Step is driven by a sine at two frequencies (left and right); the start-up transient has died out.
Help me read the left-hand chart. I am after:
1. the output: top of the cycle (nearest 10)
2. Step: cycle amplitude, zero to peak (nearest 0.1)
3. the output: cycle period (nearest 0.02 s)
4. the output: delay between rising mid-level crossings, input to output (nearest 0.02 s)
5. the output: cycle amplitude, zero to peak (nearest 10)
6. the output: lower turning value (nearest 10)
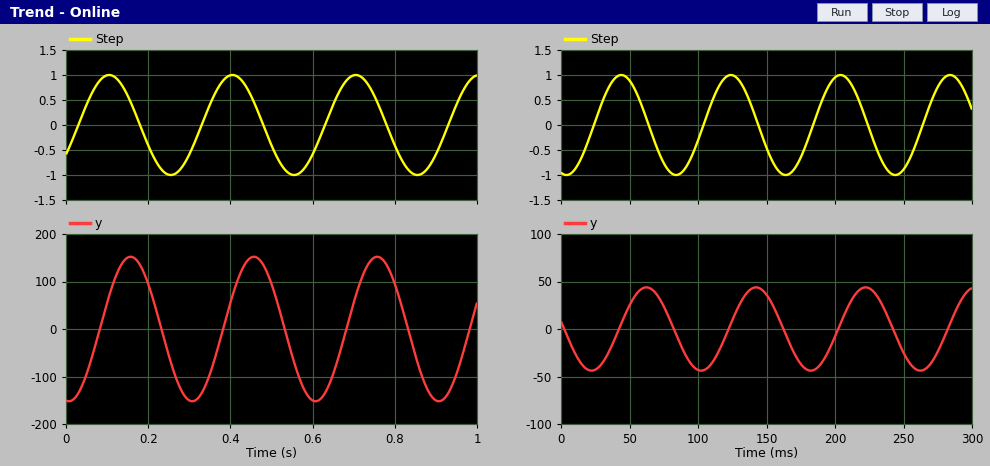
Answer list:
150
1.0
0.30 s
0.06 s
150
-150
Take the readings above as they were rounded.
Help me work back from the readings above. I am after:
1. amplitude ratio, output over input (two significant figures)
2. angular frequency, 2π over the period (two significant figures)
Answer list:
150
21 rad/s
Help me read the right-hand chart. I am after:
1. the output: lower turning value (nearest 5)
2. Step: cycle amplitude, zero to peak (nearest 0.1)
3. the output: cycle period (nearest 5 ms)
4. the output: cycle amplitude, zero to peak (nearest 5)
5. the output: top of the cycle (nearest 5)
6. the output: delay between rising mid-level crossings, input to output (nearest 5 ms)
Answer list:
-45
1.0
80 ms
45
45
20 ms
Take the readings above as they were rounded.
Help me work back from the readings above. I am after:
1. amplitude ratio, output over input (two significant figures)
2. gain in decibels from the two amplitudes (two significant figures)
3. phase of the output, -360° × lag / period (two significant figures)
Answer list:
45
33 dB
-90°
